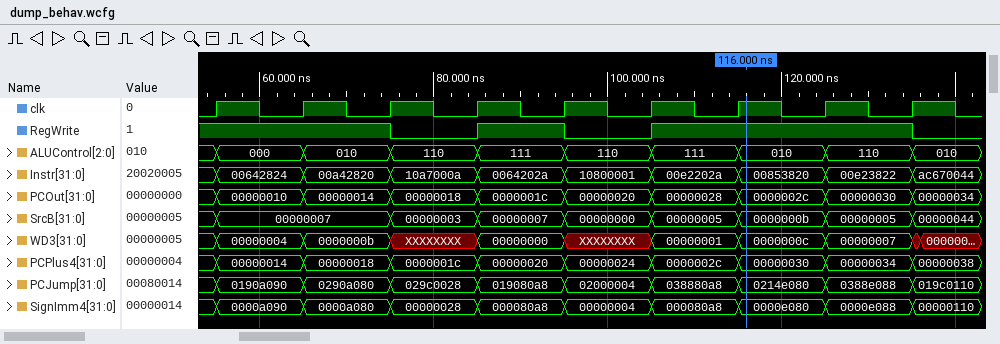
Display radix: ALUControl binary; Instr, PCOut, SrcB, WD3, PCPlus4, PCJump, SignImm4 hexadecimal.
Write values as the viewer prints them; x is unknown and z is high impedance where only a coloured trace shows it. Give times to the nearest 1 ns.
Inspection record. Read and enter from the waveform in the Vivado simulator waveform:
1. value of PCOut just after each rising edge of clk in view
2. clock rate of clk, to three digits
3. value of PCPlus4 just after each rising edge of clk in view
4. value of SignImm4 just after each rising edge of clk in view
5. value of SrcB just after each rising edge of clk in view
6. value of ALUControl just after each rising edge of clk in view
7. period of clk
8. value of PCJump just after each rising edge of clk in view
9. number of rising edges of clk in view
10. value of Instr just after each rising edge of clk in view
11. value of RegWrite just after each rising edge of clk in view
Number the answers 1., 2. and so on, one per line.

1. 00000010, 00000014, 00000018, 0000001c, 00000020, 00000028, 0000002c, 00000030, 00000034
2. 100 MHz
3. 00000014, 00000018, 0000001c, 00000020, 00000024, 0000002c, 00000030, 00000034, 00000038
4. 0000a090, 0000a080, 00000028, 000080a8, 00000004, 000080a8, 0000e080, 0000e088, 00000110
5. 00000007, 00000007, 00000003, 00000007, 00000000, 00000005, 0000000b, 00000005, 00000044
6. 000, 010, 110, 111, 110, 111, 010, 110, 010
7. 10 ns
8. 0190a090, 0290a080, 029c0028, 019080a8, 02000004, 038880a8, 0214e080, 0388e088, 019c0110
9. 9
10. 00642824, 00a42820, 10a7000a, 0064202a, 10800001, 00e2202a, 00853820, 00e23822, ac670044
11. 1 1 0 1 0 1 1 1 0
